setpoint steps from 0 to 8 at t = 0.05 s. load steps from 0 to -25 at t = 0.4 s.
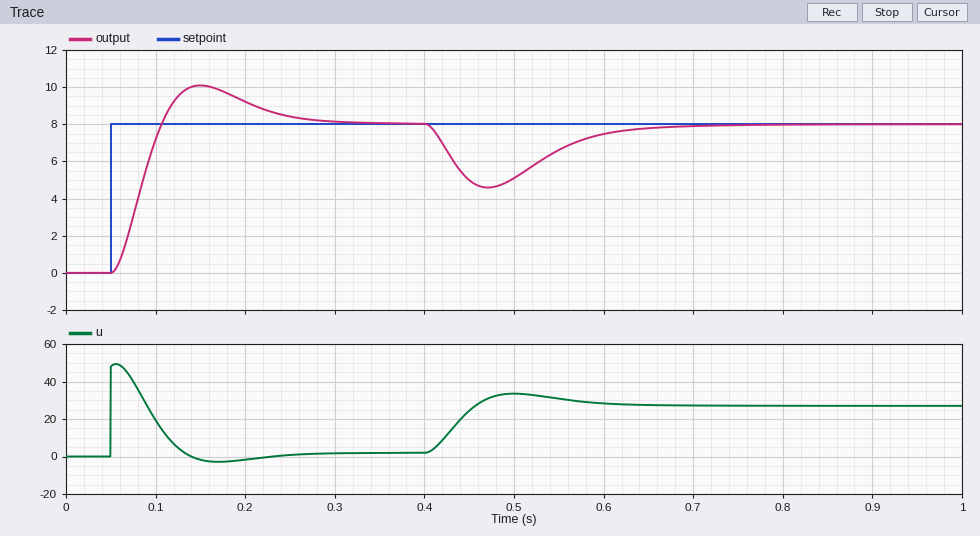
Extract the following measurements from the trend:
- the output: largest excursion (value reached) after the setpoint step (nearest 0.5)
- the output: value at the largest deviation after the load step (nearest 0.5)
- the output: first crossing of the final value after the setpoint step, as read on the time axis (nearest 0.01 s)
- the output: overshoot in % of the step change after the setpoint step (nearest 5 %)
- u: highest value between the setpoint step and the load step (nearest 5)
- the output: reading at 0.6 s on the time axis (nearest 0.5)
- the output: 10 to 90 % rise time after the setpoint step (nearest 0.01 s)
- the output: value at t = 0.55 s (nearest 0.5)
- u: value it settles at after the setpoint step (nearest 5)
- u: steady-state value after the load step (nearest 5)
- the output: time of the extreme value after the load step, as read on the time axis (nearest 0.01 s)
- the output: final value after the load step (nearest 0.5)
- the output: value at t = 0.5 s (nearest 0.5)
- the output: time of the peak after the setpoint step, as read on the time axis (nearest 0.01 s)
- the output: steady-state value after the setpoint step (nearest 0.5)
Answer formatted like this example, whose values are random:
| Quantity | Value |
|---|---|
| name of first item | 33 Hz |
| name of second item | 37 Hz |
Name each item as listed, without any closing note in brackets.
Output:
| Quantity | Value |
|---|---|
| the output: largest excursion (value reached) after the setpoint step | 10.0 |
| the output: value at the largest deviation after the load step | 4.5 |
| the output: first crossing of the final value after the setpoint step, as read on the time axis | 0.11 s |
| the output: overshoot in % of the step change after the setpoint step | 25 % |
| u: highest value between the setpoint step and the load step | 50 |
| the output: reading at 0.6 s on the time axis | 7.5 |
| the output: 10 to 90 % rise time after the setpoint step | 0.04 s |
| the output: value at t = 0.55 s | 6.5 |
| u: value it settles at after the setpoint step | 0 |
| u: steady-state value after the load step | 25 |
| the output: time of the extreme value after the load step, as read on the time axis | 0.47 s |
| the output: final value after the load step | 8.0 |
| the output: value at t = 0.5 s | 5.0 |
| the output: time of the peak after the setpoint step, as read on the time axis | 0.15 s |
| the output: steady-state value after the setpoint step | 8.0 |
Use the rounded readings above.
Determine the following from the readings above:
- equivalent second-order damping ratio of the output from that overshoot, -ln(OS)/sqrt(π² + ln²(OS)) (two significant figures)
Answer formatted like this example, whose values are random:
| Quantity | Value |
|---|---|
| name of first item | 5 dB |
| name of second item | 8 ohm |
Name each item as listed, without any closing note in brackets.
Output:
| Quantity | Value |
|---|---|
| equivalent second-order damping ratio of the output from that overshoot, -ln(OS)/sqrt(π² + ln²(OS)) | 0.40 |
